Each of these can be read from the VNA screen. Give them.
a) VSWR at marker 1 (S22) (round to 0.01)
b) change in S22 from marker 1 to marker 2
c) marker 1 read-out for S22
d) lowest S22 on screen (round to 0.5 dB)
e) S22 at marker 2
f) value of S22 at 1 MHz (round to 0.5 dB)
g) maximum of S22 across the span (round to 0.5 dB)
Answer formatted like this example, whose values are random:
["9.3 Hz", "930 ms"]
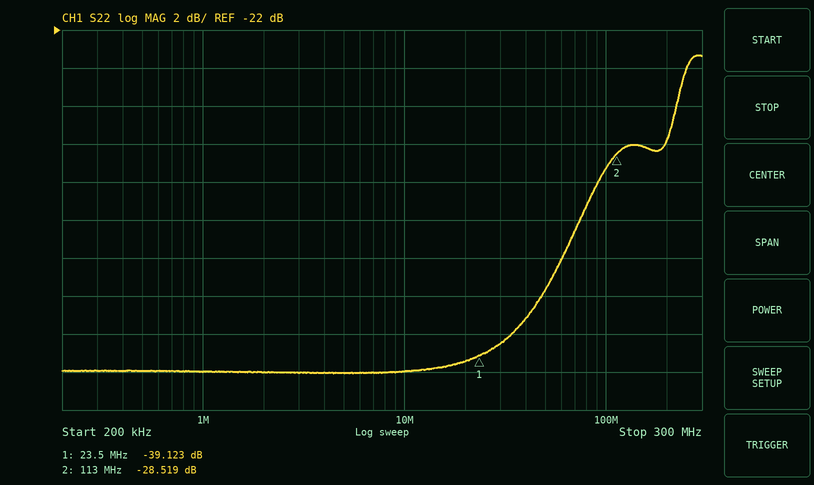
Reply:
["1.02", "10.604 dB", "-39.123 dB", "-40.0 dB", "-28.519 dB", "-40.0 dB", "-23.5 dB"]
